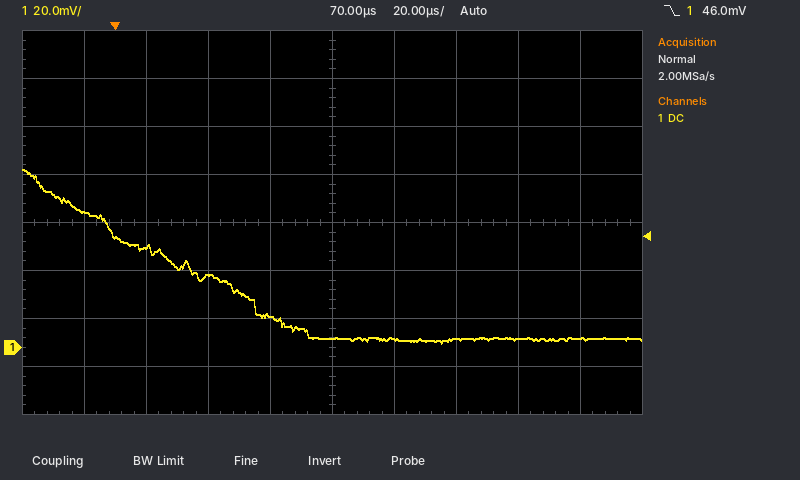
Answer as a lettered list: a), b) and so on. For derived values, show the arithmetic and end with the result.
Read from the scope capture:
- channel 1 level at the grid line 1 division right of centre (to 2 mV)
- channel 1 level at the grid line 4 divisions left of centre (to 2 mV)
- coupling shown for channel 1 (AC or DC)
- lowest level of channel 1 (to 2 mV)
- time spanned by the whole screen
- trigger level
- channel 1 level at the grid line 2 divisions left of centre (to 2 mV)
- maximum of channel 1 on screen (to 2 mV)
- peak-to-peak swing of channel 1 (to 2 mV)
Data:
a) 4 mV
b) 56 mV
c) DC
d) 2 mV
e) 200 µs
f) 46.0 mV
g) 30 mV
h) 74 mV
i) 74 mV − (2 mV) = 72 mV
